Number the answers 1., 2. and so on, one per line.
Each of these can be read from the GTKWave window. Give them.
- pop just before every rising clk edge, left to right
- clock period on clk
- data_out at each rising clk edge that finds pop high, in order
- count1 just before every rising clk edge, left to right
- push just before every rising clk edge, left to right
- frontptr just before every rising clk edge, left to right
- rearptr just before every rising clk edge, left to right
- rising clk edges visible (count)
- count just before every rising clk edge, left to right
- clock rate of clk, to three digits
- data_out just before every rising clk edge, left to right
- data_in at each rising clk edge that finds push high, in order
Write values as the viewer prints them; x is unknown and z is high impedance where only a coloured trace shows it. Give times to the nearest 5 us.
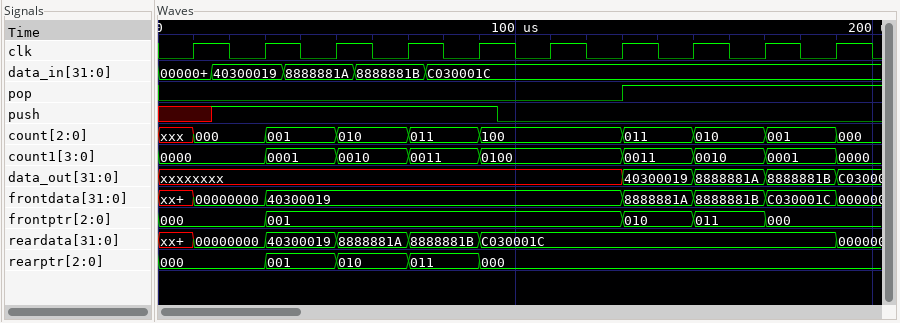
1. 0 0 0 0 0 0 0 1 1 1
2. 20 us
3. 40300019, 8888881A, 8888881B
4. 0000, 0000, 0001, 0010, 0011, 0100, 0100, 0011, 0010, 0001
5. x 1 1 1 1 0 0 0 0 0
6. 000, 000, 001, 001, 001, 001, 001, 010, 011, 000
7. 000, 000, 001, 010, 011, 000, 000, 000, 000, 000
8. 10
9. xxx, 000, 001, 010, 011, 100, 100, 011, 010, 001
10. 50.0 kHz
11. xxxxxxxx, xxxxxxxx, xxxxxxxx, xxxxxxxx, xxxxxxxx, xxxxxxxx, xxxxxxxx, 40300019, 8888881A, 8888881B
12. 40300019, 8888881A, 8888881B, C030001C
